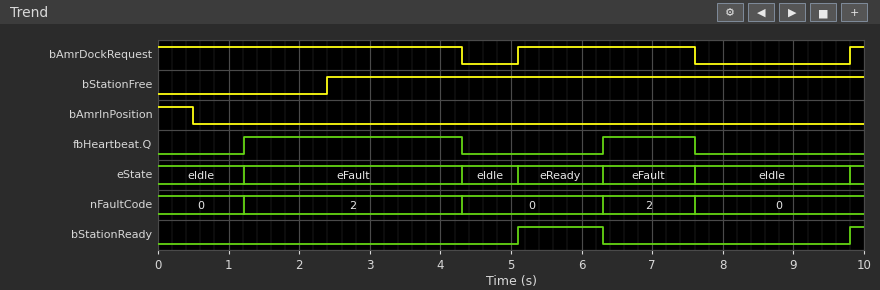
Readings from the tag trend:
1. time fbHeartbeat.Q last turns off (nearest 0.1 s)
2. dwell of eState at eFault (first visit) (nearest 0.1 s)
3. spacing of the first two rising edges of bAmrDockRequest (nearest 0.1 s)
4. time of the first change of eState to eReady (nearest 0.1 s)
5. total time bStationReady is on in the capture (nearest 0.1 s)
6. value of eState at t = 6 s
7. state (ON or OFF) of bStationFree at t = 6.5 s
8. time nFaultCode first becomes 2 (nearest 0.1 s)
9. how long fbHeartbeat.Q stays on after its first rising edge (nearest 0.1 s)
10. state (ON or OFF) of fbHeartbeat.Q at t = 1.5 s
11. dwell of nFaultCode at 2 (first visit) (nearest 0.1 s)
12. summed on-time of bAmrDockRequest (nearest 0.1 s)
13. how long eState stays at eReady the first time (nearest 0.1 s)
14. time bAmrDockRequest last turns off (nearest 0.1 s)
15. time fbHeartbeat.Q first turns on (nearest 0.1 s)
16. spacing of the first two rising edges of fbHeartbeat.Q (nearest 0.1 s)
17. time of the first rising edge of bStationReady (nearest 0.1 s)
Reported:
7.6 s
3.1 s
4.7 s
5.1 s
1.4 s
eReady
ON
1.2 s
3.1 s
ON
3.1 s
7.0 s
1.2 s
7.6 s
1.2 s
5.1 s
5.1 s
